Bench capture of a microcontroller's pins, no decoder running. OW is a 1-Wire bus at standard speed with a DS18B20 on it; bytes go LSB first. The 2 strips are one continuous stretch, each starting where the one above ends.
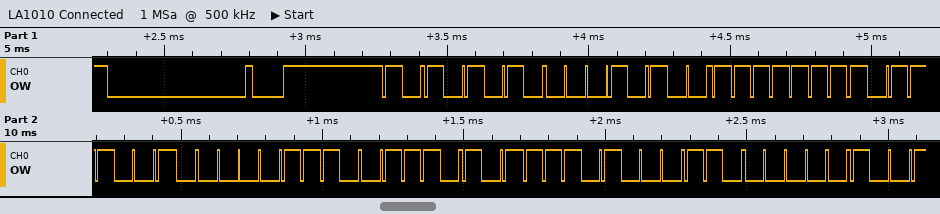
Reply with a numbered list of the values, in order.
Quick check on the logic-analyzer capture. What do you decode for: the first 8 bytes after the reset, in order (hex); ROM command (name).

1. 55 28 FF 4E 70 AE 17 03
2. Match ROM
